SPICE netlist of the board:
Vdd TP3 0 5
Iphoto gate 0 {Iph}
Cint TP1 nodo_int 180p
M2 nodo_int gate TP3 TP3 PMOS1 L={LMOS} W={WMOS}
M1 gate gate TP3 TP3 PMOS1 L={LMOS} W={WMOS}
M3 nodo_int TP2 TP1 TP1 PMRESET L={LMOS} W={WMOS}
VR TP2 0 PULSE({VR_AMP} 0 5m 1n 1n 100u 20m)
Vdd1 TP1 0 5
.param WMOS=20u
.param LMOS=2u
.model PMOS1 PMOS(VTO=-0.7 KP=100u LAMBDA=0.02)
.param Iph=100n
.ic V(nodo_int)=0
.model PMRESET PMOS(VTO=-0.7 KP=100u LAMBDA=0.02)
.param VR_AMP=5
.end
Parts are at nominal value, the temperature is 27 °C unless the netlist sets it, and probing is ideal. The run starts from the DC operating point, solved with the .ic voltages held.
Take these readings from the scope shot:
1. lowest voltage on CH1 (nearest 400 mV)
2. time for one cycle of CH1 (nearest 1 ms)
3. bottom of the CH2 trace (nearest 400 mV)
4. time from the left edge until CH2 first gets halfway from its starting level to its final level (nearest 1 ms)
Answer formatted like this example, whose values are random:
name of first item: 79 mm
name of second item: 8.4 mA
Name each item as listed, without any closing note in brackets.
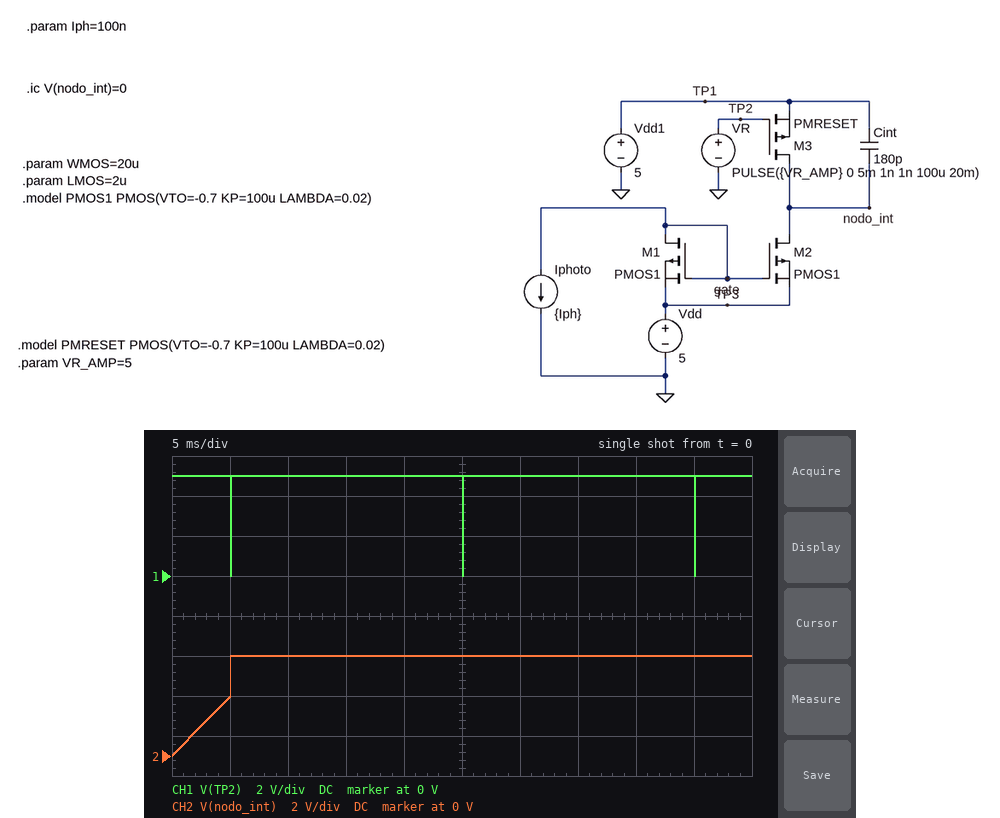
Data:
lowest voltage on CH1: 0 V
time for one cycle of CH1: 20 ms
bottom of the CH2 trace: 0 V
time from the left edge until CH2 first gets halfway from its starting level to its final level: 4 ms
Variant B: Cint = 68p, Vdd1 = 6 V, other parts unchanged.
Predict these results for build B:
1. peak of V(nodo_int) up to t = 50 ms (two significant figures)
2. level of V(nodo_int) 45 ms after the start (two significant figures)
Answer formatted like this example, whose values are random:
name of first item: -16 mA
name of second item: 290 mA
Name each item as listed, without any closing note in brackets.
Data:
peak of V(nodo_int) up to t = 50 ms: 5.7 V
level of V(nodo_int) 45 ms after the start: 5.3 V
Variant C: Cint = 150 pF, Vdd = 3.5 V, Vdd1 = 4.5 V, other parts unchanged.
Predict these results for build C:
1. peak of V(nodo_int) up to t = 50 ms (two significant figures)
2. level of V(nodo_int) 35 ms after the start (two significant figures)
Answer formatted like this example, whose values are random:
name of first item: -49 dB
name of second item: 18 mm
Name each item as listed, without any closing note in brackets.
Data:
peak of V(nodo_int) up to t = 50 ms: 4.2 V
level of V(nodo_int) 35 ms after the start: 3.5 V
